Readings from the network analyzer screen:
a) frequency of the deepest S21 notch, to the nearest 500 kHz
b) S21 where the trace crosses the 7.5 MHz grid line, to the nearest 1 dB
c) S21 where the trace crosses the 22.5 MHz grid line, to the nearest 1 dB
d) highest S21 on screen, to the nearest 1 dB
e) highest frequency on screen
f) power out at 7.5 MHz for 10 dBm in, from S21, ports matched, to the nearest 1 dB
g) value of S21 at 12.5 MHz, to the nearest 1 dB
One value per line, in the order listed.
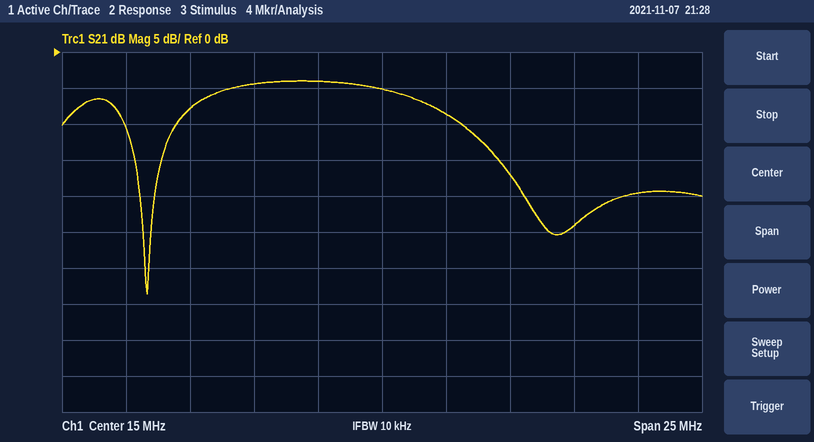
6.0 MHz
-8 dB
-24 dB
-4 dB
27.5 MHz
2 dBm
-4 dB
